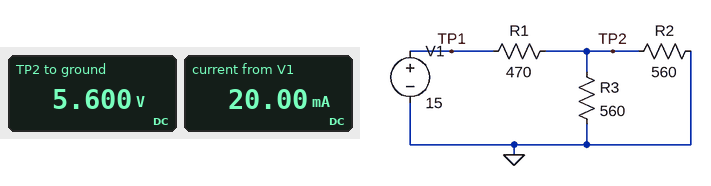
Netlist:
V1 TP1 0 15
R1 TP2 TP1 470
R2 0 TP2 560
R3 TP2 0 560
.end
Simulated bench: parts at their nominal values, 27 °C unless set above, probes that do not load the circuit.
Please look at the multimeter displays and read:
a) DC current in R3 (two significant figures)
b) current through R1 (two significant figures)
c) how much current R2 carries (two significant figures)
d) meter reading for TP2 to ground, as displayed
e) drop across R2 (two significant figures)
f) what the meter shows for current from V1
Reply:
10 mA
20 mA
10 mA
5.600 V
5.6 V
20.00 mA
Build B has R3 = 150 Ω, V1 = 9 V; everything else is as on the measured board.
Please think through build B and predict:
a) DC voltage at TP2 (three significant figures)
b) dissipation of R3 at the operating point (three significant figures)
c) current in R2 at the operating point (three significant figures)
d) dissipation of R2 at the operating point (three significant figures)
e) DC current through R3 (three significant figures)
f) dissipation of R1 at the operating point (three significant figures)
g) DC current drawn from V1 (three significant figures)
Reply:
1.81 V
21.8 mW
3.23 mA
5.85 mW
12.1 mA
110 mW
15.3 mA
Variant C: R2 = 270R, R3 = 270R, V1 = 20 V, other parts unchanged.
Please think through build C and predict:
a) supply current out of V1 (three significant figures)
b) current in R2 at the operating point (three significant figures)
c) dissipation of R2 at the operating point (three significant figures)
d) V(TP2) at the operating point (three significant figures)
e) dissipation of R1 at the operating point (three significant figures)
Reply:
33.1 mA
16.5 mA
73.8 mW
4.46 V
514 mW
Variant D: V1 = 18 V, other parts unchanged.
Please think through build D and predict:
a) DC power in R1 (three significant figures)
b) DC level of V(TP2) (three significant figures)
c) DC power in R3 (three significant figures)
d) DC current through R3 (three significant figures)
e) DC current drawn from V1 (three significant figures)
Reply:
271 mW
6.72 V
80.6 mW
12.0 mA
24.0 mA
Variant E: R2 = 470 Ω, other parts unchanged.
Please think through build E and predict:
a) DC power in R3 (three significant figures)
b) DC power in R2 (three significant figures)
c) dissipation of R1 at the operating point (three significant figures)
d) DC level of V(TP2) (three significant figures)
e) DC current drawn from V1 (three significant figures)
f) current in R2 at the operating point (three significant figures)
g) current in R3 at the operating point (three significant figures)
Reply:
49.8 mW
59.4 mW
201 mW
5.28 V
20.7 mA
11.2 mA
9.43 mA
